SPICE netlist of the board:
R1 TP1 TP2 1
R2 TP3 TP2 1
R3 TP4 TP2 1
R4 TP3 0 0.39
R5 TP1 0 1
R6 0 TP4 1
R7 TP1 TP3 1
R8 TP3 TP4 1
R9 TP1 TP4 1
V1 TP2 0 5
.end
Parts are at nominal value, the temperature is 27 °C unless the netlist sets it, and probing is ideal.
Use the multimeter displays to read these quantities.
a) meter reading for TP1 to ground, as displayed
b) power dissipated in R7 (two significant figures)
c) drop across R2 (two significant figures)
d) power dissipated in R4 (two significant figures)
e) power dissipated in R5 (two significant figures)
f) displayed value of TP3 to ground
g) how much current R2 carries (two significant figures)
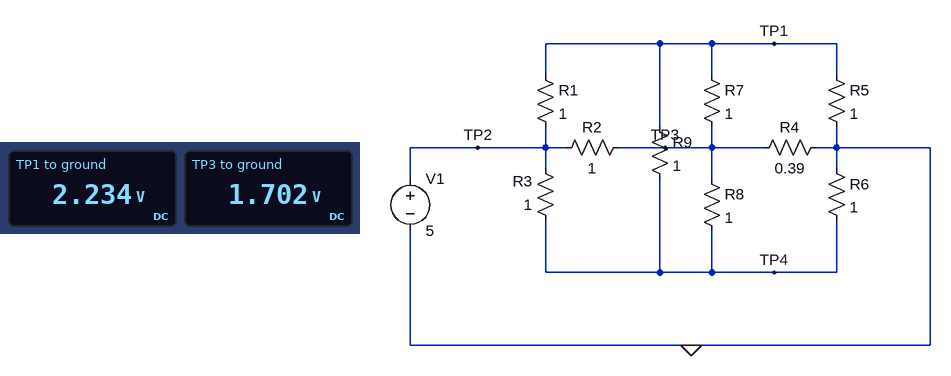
2.234 V
280 mW
3.3 V
7.4 W
5.0 W
1.702 V
3.3 A
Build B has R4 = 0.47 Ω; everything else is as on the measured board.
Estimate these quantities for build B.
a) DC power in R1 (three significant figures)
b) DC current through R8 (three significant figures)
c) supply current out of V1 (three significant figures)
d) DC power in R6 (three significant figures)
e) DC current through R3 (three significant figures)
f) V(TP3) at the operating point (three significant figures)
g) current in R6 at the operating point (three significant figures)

7.35 W
421 mA
8.55 A
5.24 W
2.71 A
1.87 V
2.29 A
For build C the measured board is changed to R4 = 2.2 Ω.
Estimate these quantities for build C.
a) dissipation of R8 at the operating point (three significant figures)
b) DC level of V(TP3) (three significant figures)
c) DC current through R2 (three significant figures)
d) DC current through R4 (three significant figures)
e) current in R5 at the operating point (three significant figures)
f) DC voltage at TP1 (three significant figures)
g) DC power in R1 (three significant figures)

106 mW
2.99 V
2.01 A
1.36 A
2.66 A
2.66 V
5.46 W
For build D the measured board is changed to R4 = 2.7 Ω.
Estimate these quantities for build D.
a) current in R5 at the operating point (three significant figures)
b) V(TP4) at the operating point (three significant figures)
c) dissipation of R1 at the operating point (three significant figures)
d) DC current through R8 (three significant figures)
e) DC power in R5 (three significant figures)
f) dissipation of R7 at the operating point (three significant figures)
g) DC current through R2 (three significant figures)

2.69 A
2.69 V
5.32 W
388 mA
7.26 W
151 mW
1.92 A
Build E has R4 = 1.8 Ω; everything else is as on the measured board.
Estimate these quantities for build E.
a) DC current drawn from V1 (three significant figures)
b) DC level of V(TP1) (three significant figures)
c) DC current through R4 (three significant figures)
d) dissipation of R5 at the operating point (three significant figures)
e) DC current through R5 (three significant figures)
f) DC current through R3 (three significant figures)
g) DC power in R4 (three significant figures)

6.86 A
2.63 V
1.60 A
6.91 W
2.63 A
2.37 A
4.62 W
